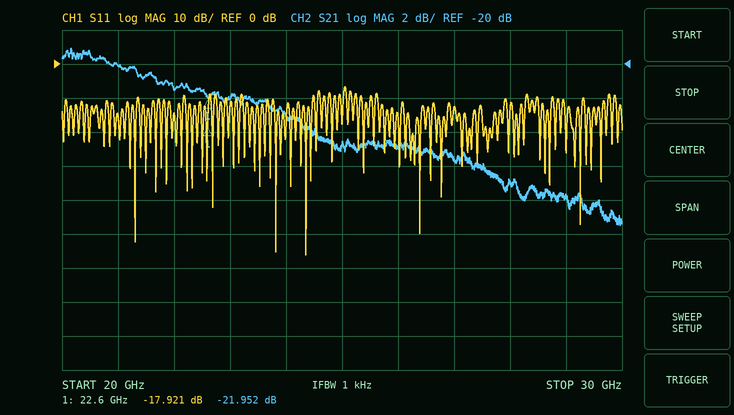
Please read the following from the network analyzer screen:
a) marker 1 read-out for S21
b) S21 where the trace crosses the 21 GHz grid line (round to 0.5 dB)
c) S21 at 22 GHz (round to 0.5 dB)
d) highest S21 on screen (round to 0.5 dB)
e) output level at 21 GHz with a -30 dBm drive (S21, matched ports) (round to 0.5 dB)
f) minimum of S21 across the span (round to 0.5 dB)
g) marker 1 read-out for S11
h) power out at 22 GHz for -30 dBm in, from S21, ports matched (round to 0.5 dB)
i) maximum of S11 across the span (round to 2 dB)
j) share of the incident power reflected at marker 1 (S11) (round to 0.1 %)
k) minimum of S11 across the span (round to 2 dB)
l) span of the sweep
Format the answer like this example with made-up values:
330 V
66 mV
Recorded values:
-21.952 dB
-20.0 dB
-21.5 dB
-19.0 dB
-50.0 dBm
-29.5 dB
-17.921 dB
-51.5 dBm
-6 dB
1.6 %
-56 dB
10 GHz
